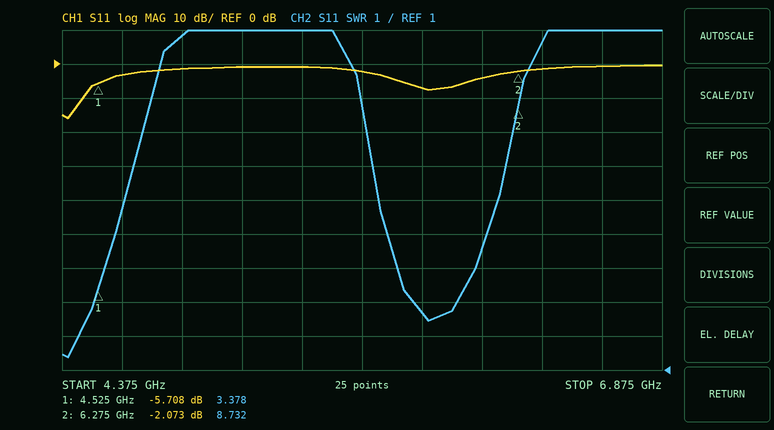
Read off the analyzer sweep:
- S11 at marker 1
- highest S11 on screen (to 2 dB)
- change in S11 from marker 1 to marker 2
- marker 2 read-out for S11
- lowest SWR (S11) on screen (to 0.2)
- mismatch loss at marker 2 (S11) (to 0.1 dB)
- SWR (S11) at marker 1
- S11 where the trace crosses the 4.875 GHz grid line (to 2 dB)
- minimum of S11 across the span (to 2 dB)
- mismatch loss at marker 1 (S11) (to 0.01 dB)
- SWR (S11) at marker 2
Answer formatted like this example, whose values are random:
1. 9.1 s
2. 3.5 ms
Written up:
1. -5.708 dB
2. 0 dB
3. 3.635 dB
4. -2.073 dB
5. 1.4
6. 4.2 dB
7. 3.378
8. -2 dB
9. -16 dB
10. 1.36 dB
11. 8.732
